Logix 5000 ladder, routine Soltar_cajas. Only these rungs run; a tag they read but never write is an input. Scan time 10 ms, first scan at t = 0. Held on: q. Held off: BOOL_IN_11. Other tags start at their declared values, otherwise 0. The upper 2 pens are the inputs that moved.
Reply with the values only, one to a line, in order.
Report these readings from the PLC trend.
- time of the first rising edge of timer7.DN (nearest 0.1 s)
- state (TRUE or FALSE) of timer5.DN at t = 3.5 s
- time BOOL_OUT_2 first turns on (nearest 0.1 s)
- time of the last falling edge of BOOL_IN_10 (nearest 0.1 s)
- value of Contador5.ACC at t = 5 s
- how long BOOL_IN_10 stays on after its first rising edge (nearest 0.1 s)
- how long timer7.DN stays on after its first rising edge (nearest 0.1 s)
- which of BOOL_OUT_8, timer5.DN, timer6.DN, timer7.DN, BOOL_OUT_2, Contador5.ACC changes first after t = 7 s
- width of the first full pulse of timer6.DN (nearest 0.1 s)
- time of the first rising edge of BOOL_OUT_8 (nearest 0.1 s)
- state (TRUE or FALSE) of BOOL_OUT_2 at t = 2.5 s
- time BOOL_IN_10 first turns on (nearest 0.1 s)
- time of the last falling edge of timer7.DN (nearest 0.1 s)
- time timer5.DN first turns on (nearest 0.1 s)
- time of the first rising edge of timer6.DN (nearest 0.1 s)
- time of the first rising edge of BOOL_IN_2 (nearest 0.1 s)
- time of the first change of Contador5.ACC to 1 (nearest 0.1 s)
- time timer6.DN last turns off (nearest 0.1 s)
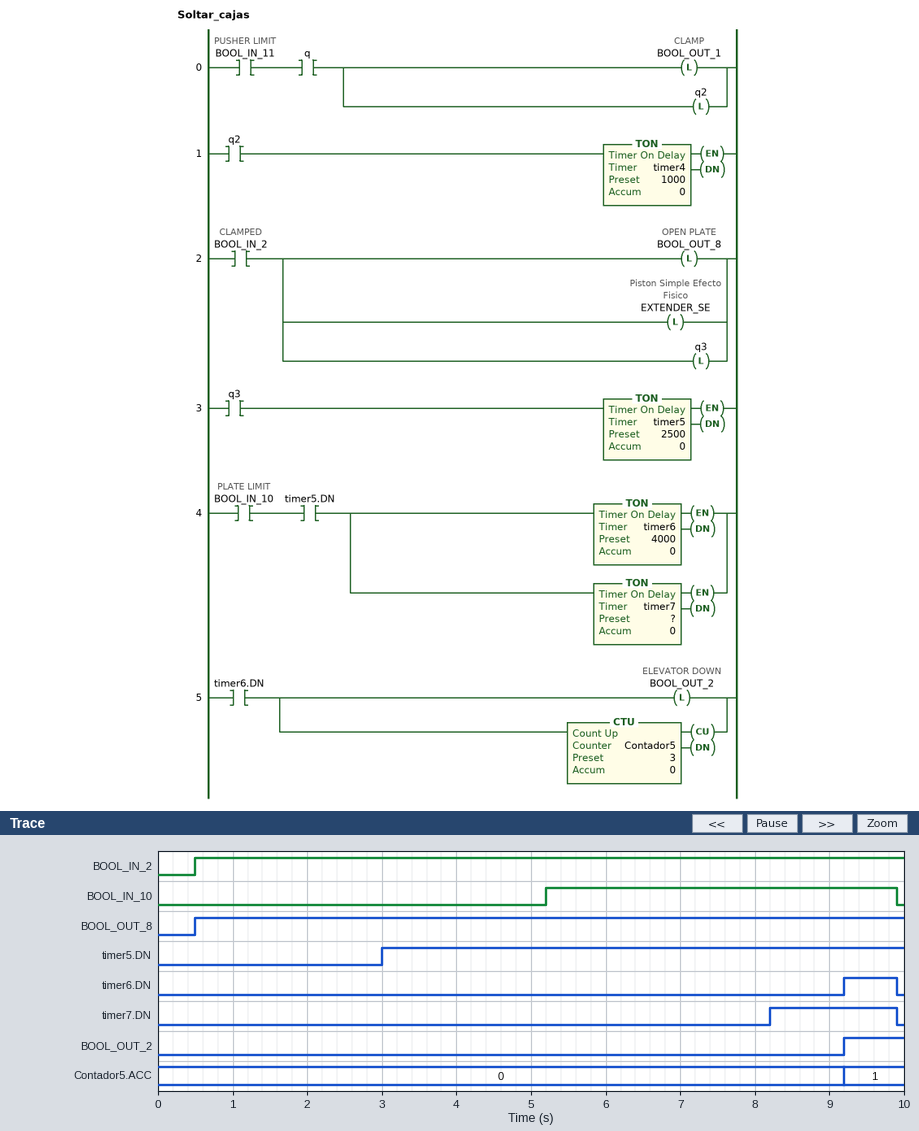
8.2 s
TRUE
9.2 s
9.9 s
0
4.7 s
1.7 s
timer7.DN
0.7 s
0.5 s
FALSE
5.2 s
9.9 s
3.0 s
9.2 s
0.5 s
9.2 s
9.9 s
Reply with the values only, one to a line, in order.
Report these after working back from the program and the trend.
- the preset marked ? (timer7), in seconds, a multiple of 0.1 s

3.0 s
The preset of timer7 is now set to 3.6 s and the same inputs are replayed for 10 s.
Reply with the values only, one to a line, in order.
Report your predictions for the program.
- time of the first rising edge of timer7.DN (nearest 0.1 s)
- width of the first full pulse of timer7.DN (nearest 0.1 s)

8.8 s
1.1 s
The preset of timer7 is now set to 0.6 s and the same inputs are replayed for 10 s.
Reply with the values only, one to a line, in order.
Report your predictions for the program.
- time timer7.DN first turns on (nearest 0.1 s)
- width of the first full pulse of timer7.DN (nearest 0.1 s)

5.8 s
4.1 s
